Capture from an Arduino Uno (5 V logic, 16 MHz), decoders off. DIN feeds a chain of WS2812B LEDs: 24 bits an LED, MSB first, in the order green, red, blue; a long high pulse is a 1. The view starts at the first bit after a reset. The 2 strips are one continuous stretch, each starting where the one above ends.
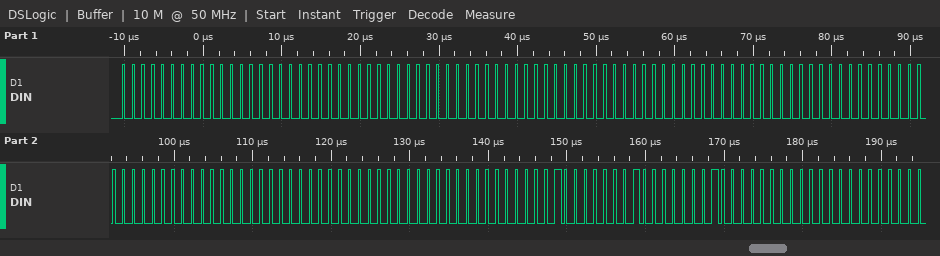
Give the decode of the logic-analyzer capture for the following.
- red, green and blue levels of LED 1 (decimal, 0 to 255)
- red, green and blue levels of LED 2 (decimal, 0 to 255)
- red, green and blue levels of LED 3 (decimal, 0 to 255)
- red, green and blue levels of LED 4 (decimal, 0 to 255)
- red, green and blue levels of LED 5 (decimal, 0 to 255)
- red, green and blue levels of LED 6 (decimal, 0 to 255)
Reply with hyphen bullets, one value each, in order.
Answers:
- 0, 0, 0
- 0, 0, 0
- 0, 0, 0
- 0, 0, 0
- 0, 0, 0
- 1, 1, 1
